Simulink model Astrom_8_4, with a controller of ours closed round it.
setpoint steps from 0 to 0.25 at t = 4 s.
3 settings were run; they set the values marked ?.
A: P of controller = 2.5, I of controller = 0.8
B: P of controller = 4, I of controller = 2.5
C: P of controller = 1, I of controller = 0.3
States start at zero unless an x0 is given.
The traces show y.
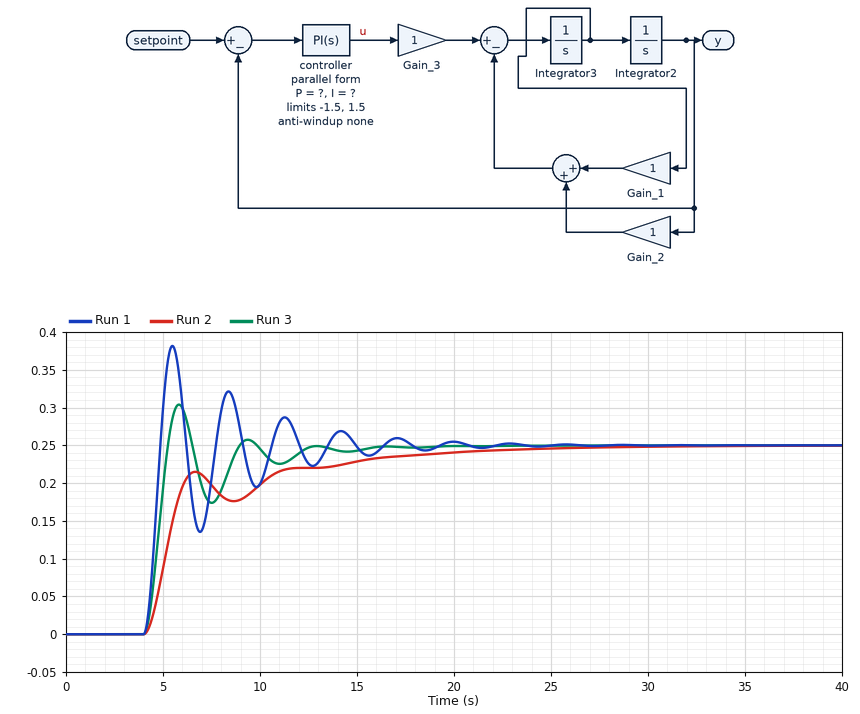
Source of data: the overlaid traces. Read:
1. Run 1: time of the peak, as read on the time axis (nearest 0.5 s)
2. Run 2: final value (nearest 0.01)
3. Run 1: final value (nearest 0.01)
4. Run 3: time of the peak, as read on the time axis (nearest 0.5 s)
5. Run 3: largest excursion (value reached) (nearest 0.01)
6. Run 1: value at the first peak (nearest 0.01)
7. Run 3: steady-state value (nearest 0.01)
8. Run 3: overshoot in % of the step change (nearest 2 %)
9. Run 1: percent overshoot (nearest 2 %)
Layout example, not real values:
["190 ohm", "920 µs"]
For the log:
["5.5 s", "0.25", "0.25", "6.0 s", "0.30", "0.38", "0.25", "22 %", "52 %"]
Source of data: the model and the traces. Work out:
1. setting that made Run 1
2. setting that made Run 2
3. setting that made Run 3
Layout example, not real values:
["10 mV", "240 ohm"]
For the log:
["B", "C", "A"]
